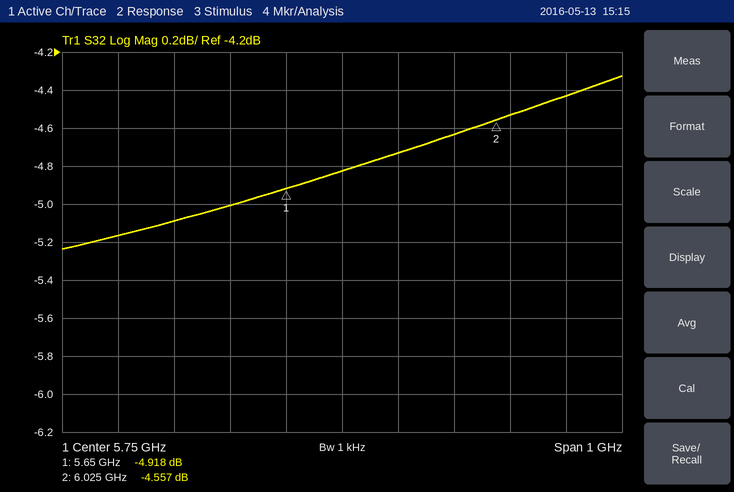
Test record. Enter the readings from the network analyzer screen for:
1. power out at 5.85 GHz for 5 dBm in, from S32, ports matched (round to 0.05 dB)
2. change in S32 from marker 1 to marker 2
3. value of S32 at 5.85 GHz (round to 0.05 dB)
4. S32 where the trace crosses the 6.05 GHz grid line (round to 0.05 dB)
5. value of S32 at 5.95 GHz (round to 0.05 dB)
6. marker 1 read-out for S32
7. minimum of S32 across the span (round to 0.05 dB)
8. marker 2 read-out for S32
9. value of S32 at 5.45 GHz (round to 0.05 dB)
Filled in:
0.25 dBm
0.361 dB
-4.75 dB
-4.55 dB
-4.65 dB
-4.918 dB
-5.25 dB
-4.557 dB
-5.10 dB
